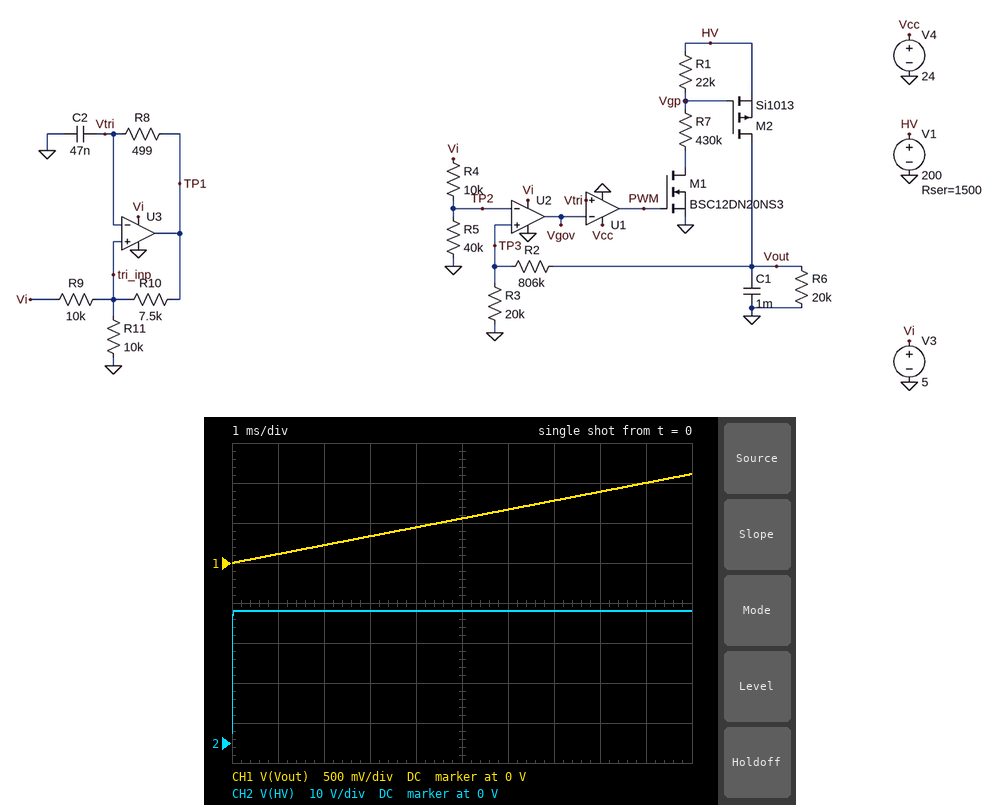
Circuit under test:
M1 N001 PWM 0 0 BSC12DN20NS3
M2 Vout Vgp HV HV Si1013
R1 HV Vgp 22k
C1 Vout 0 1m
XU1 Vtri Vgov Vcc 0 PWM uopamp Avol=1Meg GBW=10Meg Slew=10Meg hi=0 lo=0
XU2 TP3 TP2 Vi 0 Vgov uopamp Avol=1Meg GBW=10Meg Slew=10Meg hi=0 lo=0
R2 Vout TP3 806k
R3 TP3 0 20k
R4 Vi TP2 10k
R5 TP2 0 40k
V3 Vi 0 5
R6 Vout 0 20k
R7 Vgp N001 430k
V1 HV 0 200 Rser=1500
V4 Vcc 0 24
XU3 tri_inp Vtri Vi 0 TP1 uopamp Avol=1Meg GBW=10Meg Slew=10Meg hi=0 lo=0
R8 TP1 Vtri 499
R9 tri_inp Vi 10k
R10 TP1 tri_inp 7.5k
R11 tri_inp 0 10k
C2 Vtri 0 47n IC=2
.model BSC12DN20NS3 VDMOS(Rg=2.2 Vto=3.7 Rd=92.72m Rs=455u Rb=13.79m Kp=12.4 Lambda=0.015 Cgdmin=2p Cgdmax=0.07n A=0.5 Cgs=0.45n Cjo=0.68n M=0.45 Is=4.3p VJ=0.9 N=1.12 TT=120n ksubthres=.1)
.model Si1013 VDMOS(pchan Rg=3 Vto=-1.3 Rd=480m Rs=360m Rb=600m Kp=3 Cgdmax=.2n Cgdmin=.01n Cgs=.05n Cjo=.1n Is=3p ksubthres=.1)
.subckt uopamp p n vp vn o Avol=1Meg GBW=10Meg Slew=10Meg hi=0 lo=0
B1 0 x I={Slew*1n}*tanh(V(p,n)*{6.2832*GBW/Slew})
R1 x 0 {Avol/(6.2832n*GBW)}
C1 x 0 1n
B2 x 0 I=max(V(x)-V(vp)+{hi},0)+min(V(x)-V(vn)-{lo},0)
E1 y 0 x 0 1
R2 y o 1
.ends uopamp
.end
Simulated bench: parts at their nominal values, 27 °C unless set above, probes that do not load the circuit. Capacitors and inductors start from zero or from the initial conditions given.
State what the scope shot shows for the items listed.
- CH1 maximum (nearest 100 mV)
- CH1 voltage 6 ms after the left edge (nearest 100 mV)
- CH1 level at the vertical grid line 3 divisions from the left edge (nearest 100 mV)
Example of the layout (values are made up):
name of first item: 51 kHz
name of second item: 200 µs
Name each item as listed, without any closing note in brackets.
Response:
CH1 maximum: 1.1 V
CH1 voltage 6 ms after the left edge: 700 mV
CH1 level at the vertical grid line 3 divisions from the left edge: 300 mV
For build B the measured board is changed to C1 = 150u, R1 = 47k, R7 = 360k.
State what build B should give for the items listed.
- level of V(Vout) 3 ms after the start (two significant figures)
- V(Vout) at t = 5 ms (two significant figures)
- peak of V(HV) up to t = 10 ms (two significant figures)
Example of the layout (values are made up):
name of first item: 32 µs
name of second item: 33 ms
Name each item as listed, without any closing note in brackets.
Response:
level of V(Vout) 3 ms after the start: 2.5 V
V(Vout) at t = 5 ms: 4.1 V
peak of V(HV) up to t = 10 ms: 14 V
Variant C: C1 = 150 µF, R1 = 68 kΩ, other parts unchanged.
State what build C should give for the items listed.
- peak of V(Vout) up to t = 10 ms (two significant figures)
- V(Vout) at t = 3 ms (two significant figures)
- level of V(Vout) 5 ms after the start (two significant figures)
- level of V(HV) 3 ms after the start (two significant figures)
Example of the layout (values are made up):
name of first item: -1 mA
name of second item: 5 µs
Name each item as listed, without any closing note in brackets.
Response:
peak of V(Vout) up to t = 10 ms: 8.3 V
V(Vout) at t = 3 ms: 2.5 V
level of V(Vout) 5 ms after the start: 4.2 V
level of V(HV) 3 ms after the start: 12 V
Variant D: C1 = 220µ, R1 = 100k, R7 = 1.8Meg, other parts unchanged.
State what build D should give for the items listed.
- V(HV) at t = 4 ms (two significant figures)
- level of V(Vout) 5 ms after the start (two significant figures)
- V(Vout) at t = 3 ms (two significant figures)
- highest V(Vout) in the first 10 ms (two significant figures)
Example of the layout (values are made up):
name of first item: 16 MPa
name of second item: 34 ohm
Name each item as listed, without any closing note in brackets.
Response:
V(HV) at t = 4 ms: 31 V
level of V(Vout) 5 ms after the start: 2.6 V
V(Vout) at t = 3 ms: 1.5 V
highest V(Vout) in the first 10 ms: 5.1 V
